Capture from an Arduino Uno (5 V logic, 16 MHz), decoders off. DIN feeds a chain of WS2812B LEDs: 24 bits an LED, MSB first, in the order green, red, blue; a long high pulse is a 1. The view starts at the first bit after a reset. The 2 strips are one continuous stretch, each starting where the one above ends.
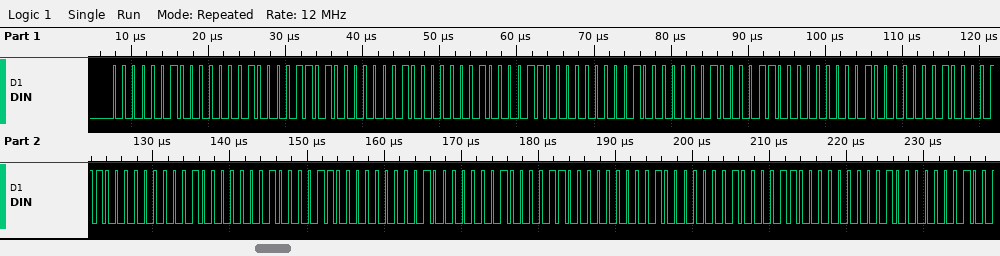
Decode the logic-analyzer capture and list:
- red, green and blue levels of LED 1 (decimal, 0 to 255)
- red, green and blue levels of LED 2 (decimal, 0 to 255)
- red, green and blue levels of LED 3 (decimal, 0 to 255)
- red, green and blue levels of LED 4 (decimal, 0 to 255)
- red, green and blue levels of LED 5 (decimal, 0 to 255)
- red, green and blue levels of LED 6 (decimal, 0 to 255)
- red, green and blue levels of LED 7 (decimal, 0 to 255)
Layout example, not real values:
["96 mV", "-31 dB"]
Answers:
["2, 2, 26", "2, 2, 24", "2, 2, 24", "2, 2, 24", "2, 2, 24", "2, 2, 24", "2, 2, 24"]
